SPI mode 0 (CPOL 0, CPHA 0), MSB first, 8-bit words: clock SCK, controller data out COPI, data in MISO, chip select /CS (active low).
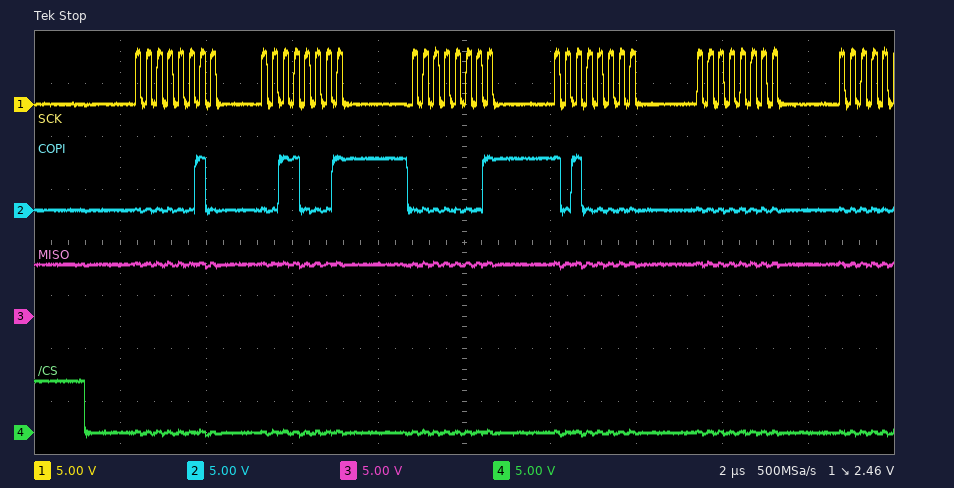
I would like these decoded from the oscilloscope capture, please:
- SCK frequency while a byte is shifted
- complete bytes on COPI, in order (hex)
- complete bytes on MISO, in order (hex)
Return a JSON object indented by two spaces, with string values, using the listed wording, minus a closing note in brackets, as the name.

{
  "SCK frequency while a byte is shifted": "4 MHz",
  "complete bytes on COPI, in order": "02 31 01 A0 00",
  "complete bytes on MISO, in order": "FF FF FF FF FF"
}
